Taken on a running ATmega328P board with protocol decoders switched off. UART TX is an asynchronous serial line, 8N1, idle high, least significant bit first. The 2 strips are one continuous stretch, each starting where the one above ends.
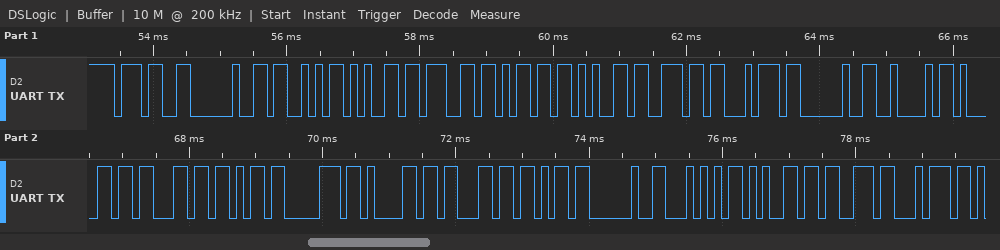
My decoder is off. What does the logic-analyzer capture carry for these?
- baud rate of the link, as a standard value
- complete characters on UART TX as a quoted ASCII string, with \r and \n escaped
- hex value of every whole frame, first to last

9600 baud
"7 Segment Backpack Test"
37 20 53 65 67 6D 65 6E 74 20 42 61 63 6B 70 61 63 6B 20 54 65 73 74
